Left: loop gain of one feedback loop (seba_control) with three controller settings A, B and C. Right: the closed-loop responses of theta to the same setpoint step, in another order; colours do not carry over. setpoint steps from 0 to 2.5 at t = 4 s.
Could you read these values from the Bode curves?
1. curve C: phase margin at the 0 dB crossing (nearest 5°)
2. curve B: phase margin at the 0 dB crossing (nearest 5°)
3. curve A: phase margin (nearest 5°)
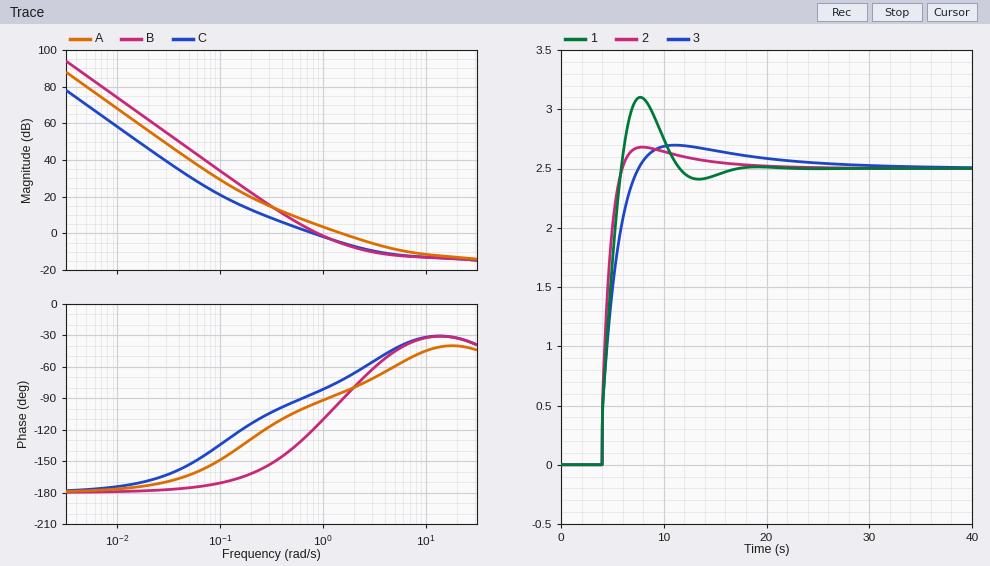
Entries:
95°
65°
95°
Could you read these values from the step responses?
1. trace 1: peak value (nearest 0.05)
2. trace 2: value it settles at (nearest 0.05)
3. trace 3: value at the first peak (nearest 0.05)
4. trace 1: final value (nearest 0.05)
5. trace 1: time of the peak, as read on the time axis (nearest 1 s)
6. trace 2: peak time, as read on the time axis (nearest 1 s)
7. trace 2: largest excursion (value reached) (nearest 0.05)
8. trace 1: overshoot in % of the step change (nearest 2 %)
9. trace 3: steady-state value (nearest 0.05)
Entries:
3.10
2.50
2.70
2.50
8 s
8 s
2.70
24 %
2.50
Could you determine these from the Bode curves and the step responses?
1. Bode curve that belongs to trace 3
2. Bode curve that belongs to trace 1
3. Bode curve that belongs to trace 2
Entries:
C
B
A
